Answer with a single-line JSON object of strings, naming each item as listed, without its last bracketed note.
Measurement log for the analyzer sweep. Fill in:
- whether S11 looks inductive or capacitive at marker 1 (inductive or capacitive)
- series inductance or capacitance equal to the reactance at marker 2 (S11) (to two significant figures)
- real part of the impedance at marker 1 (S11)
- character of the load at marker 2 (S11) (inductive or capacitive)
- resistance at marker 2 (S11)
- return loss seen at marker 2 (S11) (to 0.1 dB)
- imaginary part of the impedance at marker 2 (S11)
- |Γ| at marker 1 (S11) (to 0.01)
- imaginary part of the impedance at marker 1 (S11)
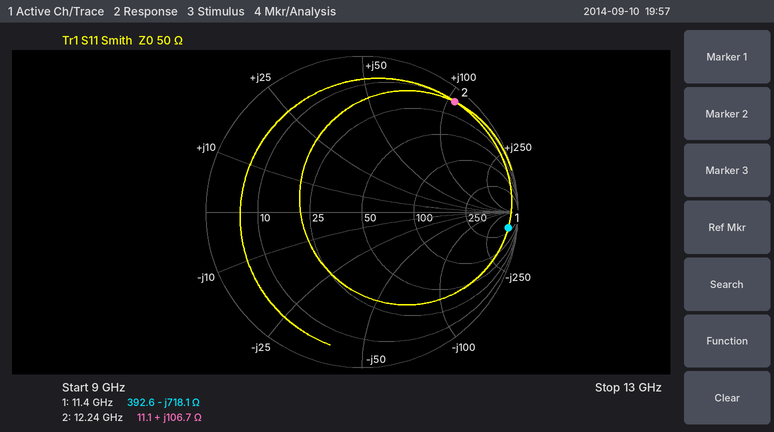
{"whether S11 looks inductive or capacitive at marker 1": "capacitive", "series inductance or capacitance equal to the reactance at marker 2 (S11)": "1.4 nH", "real part of the impedance at marker 1": "392.6 Ω", "character of the load at marker 2 (S11)": "inductive", "resistance at marker 2": "11.1 Ω", "return loss seen at marker 2 (S11)": "0.7 dB", "imaginary part of the impedance at marker 2": "+106.7 Ω", "|Γ| at marker 1 (S11)": "0.94", "imaginary part of the impedance at marker 1": "-718.1 Ω"}
